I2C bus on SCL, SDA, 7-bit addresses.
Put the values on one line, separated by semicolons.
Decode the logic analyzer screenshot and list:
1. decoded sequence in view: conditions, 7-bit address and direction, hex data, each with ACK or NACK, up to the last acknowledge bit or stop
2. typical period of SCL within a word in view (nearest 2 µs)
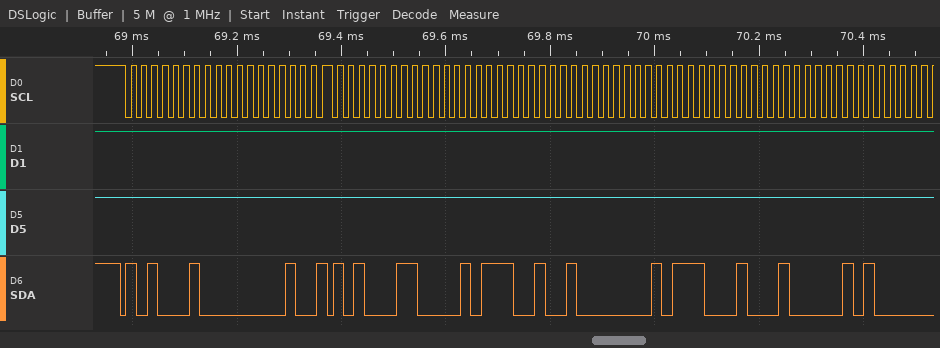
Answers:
start, address 51 write ACK, 02 ACK, repeated start, address 51 read ACK, 17 ACK, 48 ACK, 17 ACK, 22 ACK, 14 ACK; 20 µs
